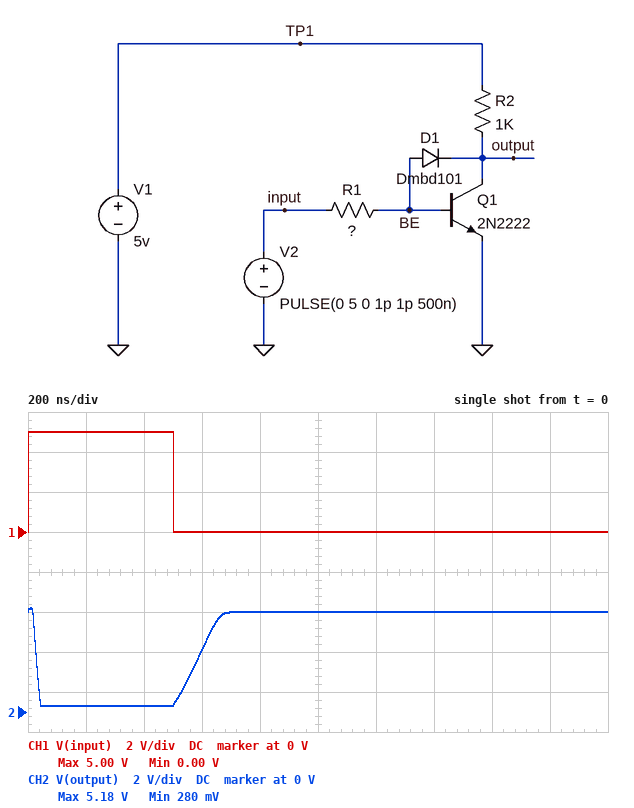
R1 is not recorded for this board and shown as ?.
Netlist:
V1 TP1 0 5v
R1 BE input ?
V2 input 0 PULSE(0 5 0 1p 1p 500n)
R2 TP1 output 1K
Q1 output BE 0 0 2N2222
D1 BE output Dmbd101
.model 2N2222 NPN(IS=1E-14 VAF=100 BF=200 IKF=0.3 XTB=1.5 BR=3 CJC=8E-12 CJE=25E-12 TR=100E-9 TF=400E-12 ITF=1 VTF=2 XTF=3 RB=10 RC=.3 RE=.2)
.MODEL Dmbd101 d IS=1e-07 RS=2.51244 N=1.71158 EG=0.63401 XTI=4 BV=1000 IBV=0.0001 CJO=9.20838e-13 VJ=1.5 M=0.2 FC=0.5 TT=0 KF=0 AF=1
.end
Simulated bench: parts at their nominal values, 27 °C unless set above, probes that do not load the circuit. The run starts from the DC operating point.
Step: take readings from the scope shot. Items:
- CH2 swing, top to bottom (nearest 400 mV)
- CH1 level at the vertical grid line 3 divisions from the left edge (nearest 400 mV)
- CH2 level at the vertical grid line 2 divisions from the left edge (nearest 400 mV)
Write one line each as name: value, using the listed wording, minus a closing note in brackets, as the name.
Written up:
CH2 swing, top to bottom: 4.8 V
CH1 level at the vertical grid line 3 divisions from the left edge: 0 V
CH2 level at the vertical grid line 2 divisions from the left edge: 400 mV
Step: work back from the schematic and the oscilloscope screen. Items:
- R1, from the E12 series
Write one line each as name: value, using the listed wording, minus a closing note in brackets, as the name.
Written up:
R1, from the E12 series: 3.3 kΩ
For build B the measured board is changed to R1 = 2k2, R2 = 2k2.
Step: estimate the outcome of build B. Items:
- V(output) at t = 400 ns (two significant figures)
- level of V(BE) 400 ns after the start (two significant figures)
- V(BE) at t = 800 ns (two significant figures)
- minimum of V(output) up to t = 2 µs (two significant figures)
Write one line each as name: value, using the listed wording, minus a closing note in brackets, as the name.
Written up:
V(output) at t = 400 ns: 250 mV
level of V(BE) 400 ns after the start: 690 mV
V(BE) at t = 800 ns: 52 mV
minimum of V(output) up to t = 2 µs: 240 mV
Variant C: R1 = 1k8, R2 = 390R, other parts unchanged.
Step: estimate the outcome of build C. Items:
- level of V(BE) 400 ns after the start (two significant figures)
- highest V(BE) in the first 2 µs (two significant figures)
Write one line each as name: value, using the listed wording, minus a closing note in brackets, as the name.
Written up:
level of V(BE) 400 ns after the start: 730 mV
highest V(BE) in the first 2 µs: 750 mV
